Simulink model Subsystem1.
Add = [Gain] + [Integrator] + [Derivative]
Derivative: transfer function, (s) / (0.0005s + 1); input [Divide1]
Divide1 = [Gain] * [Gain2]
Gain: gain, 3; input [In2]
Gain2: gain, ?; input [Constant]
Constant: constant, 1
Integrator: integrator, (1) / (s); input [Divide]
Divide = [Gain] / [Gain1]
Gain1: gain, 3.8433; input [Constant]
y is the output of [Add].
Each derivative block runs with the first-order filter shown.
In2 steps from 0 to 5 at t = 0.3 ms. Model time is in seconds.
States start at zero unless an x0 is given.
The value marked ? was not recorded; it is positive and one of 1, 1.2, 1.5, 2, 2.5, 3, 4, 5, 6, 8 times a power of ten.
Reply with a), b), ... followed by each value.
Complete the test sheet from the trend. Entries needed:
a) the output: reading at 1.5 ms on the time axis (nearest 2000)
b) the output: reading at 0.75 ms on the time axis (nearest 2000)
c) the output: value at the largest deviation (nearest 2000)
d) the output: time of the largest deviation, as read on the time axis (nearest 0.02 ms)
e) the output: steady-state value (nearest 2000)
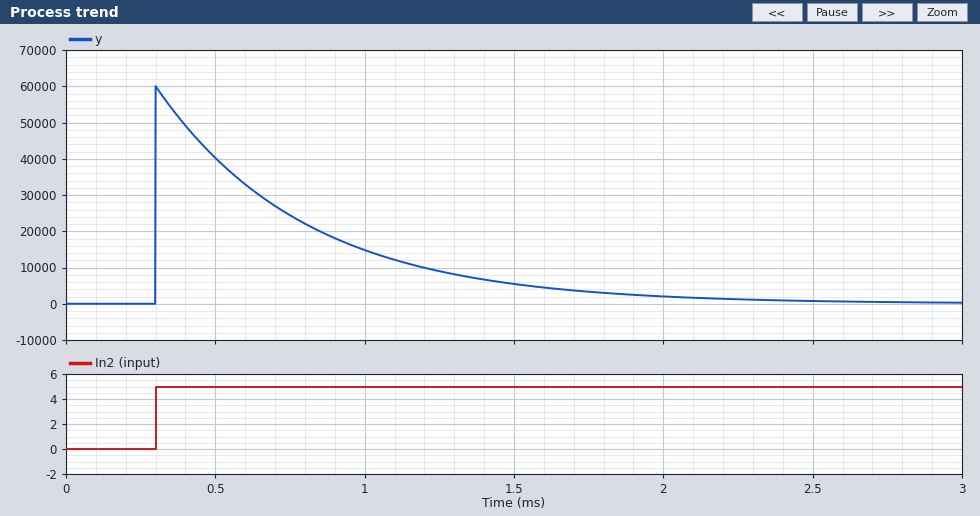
a) 6000
b) 24000
c) 60000
d) 0.30 ms
e) 0
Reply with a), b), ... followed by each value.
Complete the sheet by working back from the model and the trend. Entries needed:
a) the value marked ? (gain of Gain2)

a) 2
